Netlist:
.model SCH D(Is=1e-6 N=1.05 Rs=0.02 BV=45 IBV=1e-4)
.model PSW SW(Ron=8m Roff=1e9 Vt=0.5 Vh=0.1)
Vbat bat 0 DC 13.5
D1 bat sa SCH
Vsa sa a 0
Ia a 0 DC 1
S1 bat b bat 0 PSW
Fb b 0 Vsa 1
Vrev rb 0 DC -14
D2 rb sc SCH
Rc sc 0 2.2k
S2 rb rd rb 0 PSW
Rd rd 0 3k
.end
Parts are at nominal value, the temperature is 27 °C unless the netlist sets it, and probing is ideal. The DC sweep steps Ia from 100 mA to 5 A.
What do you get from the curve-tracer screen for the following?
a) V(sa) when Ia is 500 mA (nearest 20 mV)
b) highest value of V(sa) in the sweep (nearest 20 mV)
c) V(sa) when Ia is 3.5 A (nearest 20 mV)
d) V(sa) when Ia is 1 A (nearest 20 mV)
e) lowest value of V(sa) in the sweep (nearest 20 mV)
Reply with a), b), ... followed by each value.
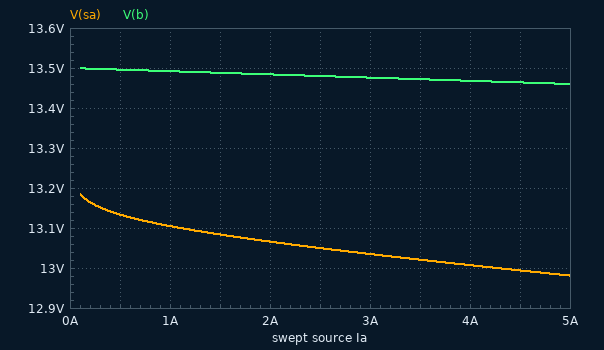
a) 13.14 V
b) 13.18 V
c) 13.02 V
d) 13.10 V
e) 12.98 V
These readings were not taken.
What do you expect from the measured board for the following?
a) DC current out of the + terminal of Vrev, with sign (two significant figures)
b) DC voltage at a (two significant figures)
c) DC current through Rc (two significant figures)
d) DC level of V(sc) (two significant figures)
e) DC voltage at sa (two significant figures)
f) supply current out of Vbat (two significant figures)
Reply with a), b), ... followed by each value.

a) -1.0 µA
b) 13 V
c) 1.0 µA
d) -2.2 mV
e) 13 V
f) 2.0 A
